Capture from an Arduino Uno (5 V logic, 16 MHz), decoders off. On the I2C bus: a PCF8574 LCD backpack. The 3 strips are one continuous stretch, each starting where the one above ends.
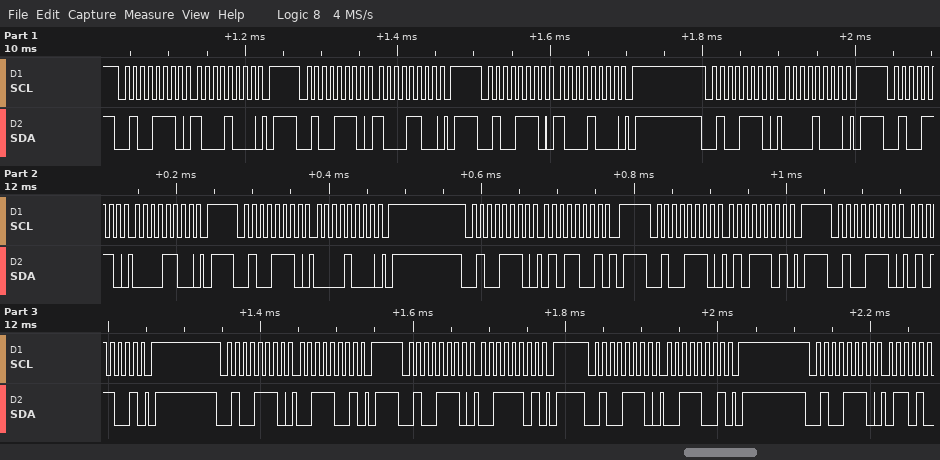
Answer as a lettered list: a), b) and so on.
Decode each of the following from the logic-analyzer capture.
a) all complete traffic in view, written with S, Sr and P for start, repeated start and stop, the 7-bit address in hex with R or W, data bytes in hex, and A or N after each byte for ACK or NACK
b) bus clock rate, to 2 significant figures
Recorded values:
a) S 27W A 88 A P S 27W A 8C A P S 27W A 88 A P S 27W A 08 A P S 27W A 0C A P S 27W A 08 A P S 27W A 59 A P S 27W A 5D A P S 27W A 59 A P S 27W A 39 A P S 27W A 3D A P S 27W A 39 A P S 27W A
b) 100 kHz
